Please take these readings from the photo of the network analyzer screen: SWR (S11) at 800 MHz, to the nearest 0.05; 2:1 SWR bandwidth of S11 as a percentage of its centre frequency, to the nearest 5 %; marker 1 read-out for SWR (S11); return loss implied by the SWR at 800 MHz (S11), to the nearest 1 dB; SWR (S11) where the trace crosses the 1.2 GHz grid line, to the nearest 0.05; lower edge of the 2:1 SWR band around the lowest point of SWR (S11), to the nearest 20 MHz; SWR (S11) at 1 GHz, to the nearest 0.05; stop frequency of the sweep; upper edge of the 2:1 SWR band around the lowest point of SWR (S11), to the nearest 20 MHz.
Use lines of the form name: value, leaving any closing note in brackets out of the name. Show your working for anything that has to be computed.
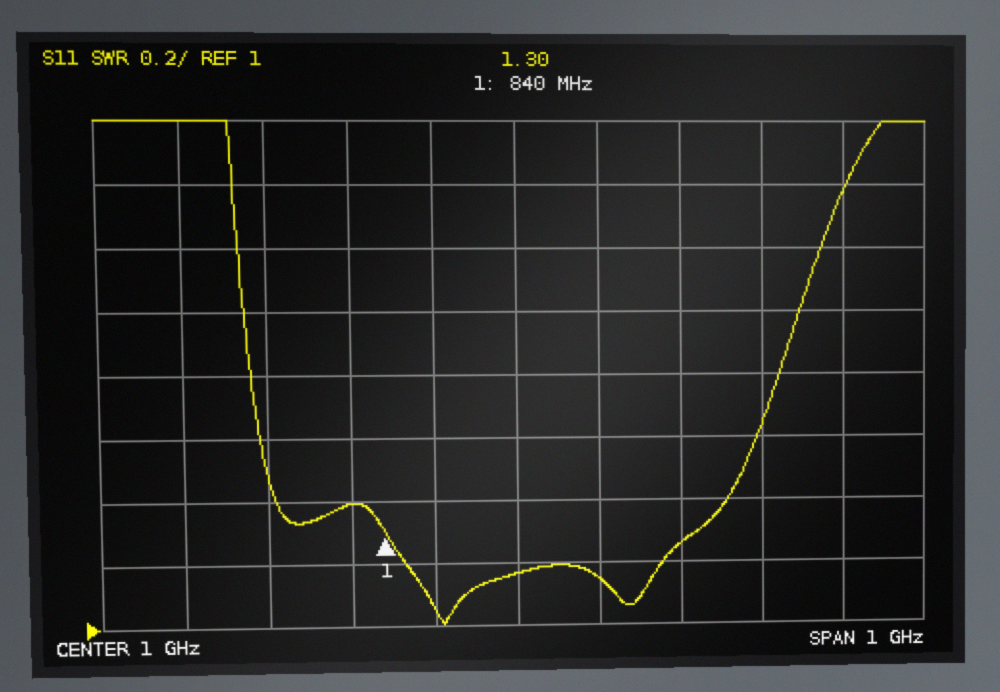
SWR (S11) at 800 MHz, to the nearest 0.05: 1.40
2:1 SWR bandwidth of S11 as a percentage of its centre frequency, to the nearest 5 %: 660 MHz / 1.01 GHz ≈ 65 %
marker 1 read-out for SWR: 1.30
return loss implied by the SWR at 800 MHz (S11), to the nearest 1 dB: −20 log10((1.4 − 1)/(1.4 + 1)) ≈ 16 dB
SWR (S11) where the trace crosses the 1.2 GHz grid line, to the nearest 0.05: 1.25
lower edge of the 2:1 SWR band around the lowest point of SWR (S11), to the nearest 20 MHz: 680 MHz
SWR (S11) at 1 GHz, to the nearest 0.05: 1.15
stop frequency of the sweep: 1.5 GHz
upper edge of the 2:1 SWR band around the lowest point of SWR (S11), to the nearest 20 MHz: 1.34 GHz
